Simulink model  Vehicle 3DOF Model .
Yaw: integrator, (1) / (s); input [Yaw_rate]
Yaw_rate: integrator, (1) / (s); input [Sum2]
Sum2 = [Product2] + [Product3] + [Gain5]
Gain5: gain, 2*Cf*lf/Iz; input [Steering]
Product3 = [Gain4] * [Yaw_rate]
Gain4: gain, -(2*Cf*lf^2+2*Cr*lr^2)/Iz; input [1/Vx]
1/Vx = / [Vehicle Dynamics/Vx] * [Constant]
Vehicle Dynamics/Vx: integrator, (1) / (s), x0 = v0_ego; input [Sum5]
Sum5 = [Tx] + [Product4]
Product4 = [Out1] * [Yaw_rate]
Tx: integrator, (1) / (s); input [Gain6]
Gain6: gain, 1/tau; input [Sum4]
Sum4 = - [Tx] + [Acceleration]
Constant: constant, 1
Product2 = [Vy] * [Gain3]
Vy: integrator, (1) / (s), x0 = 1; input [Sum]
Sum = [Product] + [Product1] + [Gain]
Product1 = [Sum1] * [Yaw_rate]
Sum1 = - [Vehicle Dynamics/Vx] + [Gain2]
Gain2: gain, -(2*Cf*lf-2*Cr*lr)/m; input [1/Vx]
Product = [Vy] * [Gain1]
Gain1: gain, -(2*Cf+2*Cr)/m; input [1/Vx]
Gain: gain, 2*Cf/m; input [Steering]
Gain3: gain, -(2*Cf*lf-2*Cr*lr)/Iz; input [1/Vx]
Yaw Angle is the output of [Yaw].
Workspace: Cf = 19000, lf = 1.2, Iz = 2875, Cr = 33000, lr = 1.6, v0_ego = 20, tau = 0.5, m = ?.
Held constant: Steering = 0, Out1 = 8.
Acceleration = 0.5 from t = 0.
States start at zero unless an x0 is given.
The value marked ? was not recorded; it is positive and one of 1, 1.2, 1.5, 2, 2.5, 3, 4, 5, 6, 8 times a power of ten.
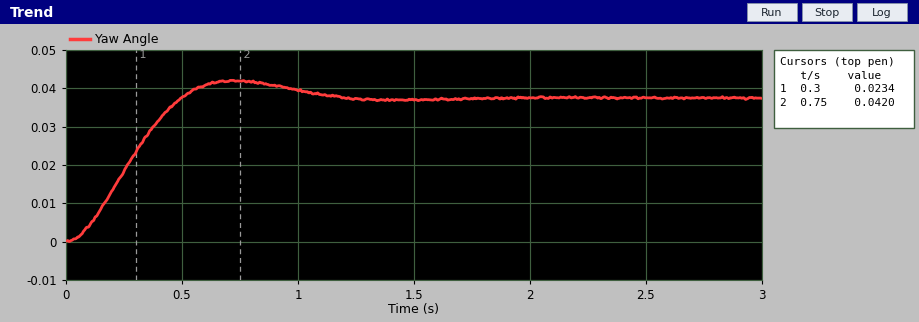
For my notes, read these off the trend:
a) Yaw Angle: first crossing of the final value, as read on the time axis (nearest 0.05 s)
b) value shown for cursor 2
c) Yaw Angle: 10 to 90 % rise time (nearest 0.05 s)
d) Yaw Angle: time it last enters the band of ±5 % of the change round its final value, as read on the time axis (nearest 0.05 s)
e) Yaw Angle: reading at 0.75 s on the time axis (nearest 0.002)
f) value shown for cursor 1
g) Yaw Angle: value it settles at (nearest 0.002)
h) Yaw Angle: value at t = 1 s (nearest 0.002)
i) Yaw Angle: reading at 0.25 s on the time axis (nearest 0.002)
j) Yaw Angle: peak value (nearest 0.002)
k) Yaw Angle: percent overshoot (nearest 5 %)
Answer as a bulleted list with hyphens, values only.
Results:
- 0.50 s
- 0.0420
- 0.35 s
- 1.00 s
- 0.042
- 0.0234
- 0.038
- 0.040
- 0.018
- 0.042
- 10 %
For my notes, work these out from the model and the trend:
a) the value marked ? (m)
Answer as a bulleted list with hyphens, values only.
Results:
- 2500
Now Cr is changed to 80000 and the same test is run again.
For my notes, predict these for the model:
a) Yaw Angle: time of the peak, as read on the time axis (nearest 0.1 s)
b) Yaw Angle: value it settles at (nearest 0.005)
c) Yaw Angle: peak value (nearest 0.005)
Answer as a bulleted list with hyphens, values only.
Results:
- 0.4 s
- 0.040
- 0.045
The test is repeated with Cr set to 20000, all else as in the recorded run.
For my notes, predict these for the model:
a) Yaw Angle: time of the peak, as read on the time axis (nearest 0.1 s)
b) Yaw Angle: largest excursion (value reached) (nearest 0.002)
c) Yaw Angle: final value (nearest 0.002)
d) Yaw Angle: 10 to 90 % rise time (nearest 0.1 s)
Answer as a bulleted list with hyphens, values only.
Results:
- 1.3 s
- 0.032
- 0.030
- 0.6 s
